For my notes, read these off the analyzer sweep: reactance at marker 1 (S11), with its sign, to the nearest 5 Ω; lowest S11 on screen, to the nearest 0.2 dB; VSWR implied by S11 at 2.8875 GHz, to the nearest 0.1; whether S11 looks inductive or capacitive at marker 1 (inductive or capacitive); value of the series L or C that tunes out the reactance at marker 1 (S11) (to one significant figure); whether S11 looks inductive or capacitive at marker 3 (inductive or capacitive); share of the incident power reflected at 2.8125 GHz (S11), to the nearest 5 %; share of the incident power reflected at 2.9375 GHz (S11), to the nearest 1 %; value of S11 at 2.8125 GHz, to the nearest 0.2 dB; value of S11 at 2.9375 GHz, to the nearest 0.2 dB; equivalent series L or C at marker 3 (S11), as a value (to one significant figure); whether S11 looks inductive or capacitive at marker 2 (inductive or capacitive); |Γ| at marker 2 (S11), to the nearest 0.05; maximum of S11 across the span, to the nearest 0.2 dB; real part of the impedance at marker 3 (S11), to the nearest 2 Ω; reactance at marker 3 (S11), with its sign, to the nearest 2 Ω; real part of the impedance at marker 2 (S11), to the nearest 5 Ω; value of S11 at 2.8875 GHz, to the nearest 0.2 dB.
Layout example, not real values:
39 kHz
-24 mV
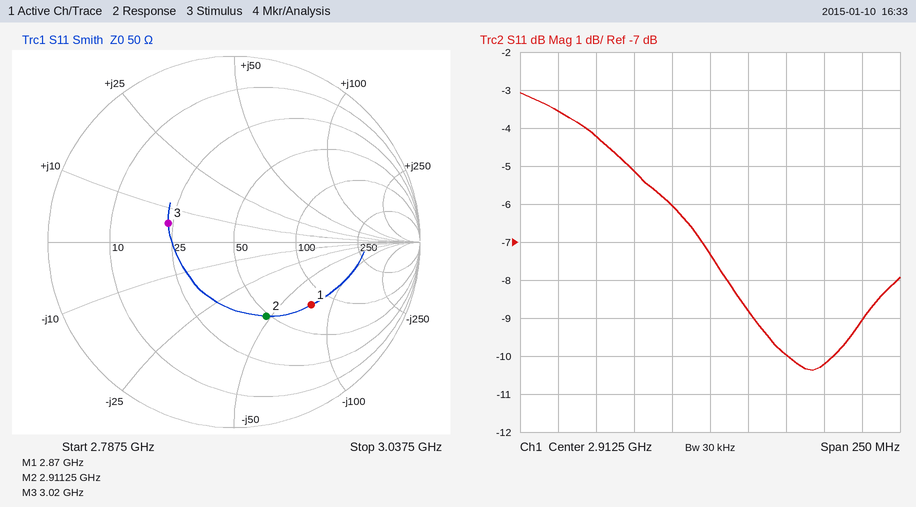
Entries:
-75 Ω
-10.4 dB
3.0
capacitive
4 nH
inductive
45 %
13 %
-3.6 dB
-8.8 dB
300 pH
capacitive
0.45
-3.0 dB
24 Ω
+6 Ω
50 Ω
-6.0 dB
